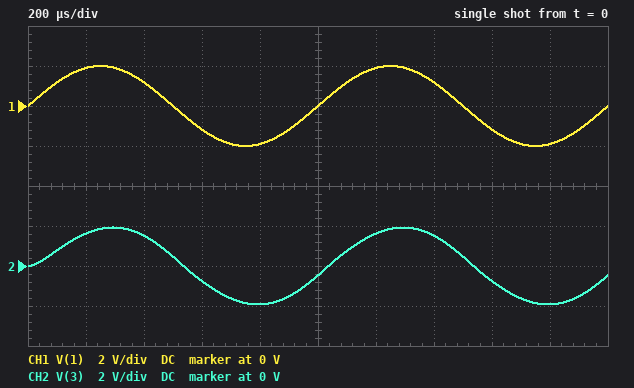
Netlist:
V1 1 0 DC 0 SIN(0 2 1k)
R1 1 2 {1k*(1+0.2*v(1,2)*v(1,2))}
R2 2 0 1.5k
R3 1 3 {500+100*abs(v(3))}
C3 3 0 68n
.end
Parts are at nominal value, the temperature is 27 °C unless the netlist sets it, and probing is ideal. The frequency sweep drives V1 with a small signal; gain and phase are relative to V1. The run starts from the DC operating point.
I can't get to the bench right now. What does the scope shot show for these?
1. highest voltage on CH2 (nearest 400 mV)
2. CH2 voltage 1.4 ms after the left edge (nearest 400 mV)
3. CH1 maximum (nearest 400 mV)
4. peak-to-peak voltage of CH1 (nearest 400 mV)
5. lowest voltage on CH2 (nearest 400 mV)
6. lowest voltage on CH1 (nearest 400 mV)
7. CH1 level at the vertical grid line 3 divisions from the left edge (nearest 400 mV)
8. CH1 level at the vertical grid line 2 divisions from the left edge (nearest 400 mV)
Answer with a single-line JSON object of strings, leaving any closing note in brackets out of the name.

{"highest voltage on CH2": "2.0 V", "CH2 voltage 1.4 ms after the left edge": "1.6 V", "CH1 maximum": "2.0 V", "peak-to-peak voltage of CH1": "4.0 V", "lowest voltage on CH2": "-2.0 V", "lowest voltage on CH1": "-2.0 V", "CH1 level at the vertical grid line 3 divisions from the left edge": "-1.2 V", "CH1 level at the vertical grid line 2 divisions from the left edge": "1.2 V"}
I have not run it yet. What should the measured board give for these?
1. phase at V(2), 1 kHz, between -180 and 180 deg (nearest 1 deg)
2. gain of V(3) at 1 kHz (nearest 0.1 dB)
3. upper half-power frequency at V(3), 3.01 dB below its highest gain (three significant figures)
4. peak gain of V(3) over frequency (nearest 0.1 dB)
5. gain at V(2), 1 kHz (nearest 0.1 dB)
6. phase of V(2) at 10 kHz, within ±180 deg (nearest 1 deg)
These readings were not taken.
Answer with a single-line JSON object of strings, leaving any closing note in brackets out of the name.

{"phase at V(2), 1 kHz, between -180 and 180 deg": "0 deg", "gain of V(3) at 1 kHz": "-0.2 dB", "upper half-power frequency at V(3), 3.01 dB below its highest gain": "4.68 kHz", "peak gain of V(3) over frequency": "0 dB", "gain at V(2), 1 kHz": "-4.4 dB", "phase of V(2) at 10 kHz, within ±180 deg": "0 deg"}
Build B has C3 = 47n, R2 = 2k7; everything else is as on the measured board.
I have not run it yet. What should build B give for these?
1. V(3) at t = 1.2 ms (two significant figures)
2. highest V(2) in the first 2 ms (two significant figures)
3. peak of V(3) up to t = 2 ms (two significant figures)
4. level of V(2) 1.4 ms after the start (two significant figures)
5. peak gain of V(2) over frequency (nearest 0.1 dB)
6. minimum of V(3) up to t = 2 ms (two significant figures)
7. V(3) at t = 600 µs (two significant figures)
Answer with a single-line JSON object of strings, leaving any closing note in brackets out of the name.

{"V(3) at t = 1.2 ms": "1.7 V", "highest V(2) in the first 2 ms": "1.4 V", "peak of V(3) up to t = 2 ms": "2.0 V", "level of V(2) 1.4 ms after the start": "850 mV", "peak gain of V(2) over frequency": "-2.7 dB", "minimum of V(3) up to t = 2 ms": "-2.0 V", "V(3) at t = 600 µs": "-880 mV"}
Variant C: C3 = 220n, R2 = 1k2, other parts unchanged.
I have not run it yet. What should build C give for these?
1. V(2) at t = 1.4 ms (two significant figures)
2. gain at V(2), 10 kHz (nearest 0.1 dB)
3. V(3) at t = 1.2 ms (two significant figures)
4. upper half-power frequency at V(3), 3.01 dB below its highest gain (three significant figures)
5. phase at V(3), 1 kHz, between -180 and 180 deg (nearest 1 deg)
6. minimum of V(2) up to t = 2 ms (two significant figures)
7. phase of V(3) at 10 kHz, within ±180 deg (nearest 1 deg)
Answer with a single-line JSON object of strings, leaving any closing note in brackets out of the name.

{"V(2) at t = 1.4 ms": "620 mV", "gain at V(2), 10 kHz": "-5.3 dB", "V(3) at t = 1.2 ms": "900 mV", "upper half-power frequency at V(3), 3.01 dB below its highest gain": "1.45 kHz", "phase at V(3), 1 kHz, between -180 and 180 deg": "-35 deg", "minimum of V(2) up to t = 2 ms": "-1.0 V", "phase of V(3) at 10 kHz, within ±180 deg": "-82 deg"}
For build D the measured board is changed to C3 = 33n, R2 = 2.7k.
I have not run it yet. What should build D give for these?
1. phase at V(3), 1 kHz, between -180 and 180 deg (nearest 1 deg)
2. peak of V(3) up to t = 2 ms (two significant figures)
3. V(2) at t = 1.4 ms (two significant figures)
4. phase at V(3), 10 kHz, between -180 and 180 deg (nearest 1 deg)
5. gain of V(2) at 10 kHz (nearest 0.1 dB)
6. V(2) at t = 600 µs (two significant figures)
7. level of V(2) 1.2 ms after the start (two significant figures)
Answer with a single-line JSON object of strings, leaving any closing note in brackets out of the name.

{"phase at V(3), 1 kHz, between -180 and 180 deg": "-6 deg", "peak of V(3) up to t = 2 ms": "2.0 V", "V(2) at t = 1.4 ms": "850 mV", "phase at V(3), 10 kHz, between -180 and 180 deg": "-46 deg", "gain of V(2) at 10 kHz": "-2.7 dB", "V(2) at t = 600 µs": "-850 mV", "level of V(2) 1.2 ms after the start": "1.4 V"}
